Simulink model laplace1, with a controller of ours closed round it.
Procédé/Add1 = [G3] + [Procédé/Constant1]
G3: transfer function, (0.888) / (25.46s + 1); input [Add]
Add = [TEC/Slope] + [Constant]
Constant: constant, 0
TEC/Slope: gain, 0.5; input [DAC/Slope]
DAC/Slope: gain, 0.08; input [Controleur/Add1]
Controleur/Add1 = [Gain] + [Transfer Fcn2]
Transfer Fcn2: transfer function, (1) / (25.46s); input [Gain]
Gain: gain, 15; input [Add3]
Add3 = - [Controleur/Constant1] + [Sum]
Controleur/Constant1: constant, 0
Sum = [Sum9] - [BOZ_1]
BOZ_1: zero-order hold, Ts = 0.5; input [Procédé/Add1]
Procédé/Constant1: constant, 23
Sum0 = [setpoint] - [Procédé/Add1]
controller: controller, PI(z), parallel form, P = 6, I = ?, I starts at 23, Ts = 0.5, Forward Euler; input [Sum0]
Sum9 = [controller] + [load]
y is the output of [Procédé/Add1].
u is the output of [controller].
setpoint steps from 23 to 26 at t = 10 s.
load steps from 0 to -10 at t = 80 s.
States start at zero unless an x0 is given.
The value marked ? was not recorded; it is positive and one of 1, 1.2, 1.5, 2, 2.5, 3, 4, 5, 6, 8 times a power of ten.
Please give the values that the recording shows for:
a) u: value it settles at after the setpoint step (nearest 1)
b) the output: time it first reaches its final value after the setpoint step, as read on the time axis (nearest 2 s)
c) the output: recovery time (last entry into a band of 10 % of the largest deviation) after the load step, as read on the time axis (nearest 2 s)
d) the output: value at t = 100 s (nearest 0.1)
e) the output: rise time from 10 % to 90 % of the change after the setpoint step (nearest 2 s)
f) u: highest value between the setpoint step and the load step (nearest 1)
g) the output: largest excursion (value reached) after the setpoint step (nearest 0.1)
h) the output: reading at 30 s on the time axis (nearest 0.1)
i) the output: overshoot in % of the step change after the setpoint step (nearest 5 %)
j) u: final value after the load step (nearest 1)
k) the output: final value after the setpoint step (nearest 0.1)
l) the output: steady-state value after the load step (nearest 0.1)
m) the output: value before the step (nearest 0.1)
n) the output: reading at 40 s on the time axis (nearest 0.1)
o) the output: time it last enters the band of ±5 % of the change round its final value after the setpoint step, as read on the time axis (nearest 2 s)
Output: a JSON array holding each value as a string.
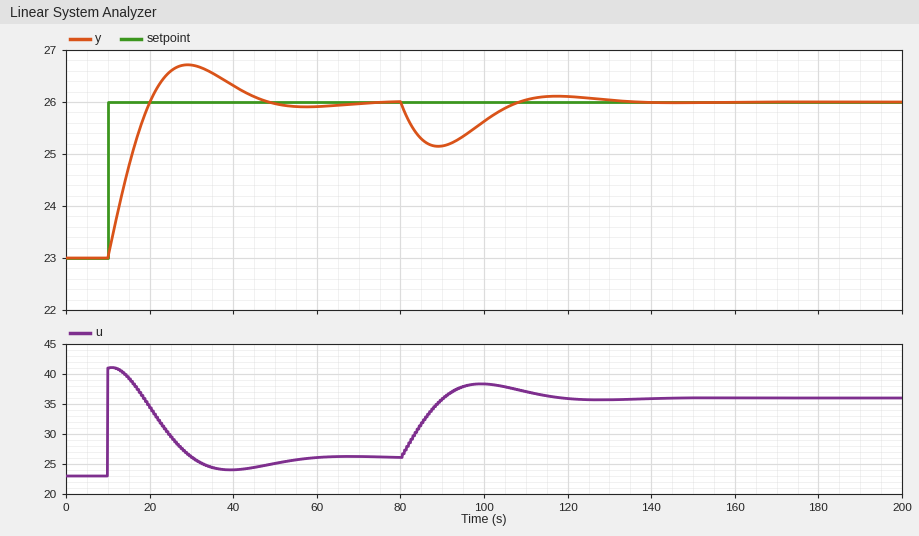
["26", "20 s", "124 s", "25.6", "8 s", "41", "26.7", "26.7", "25 %", "36", "26.0", "26.0", "23.0", "26.3", "44 s"]
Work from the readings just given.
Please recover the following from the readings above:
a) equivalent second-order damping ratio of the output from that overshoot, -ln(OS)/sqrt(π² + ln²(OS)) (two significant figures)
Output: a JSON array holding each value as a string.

["0.40"]
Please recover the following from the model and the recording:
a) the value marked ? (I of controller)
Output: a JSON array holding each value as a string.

["0.8"]
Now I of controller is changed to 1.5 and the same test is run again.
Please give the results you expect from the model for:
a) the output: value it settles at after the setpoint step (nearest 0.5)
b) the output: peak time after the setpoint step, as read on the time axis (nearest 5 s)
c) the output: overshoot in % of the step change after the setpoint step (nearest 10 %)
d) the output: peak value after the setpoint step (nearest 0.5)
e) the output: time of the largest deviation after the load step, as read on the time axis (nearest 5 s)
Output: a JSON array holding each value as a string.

["26.0", "25 s", "40 %", "27.0", "85 s"]
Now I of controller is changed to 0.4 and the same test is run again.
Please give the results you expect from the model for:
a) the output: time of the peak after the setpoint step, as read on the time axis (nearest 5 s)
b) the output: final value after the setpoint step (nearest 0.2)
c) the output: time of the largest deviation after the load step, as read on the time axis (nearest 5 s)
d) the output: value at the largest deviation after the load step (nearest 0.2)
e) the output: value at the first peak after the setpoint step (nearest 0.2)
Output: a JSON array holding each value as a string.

["35 s", "26.0", "90 s", "25.0", "26.4"]
